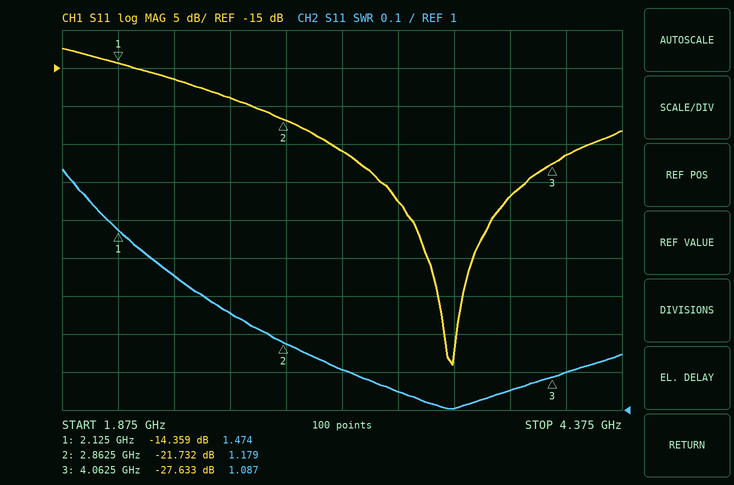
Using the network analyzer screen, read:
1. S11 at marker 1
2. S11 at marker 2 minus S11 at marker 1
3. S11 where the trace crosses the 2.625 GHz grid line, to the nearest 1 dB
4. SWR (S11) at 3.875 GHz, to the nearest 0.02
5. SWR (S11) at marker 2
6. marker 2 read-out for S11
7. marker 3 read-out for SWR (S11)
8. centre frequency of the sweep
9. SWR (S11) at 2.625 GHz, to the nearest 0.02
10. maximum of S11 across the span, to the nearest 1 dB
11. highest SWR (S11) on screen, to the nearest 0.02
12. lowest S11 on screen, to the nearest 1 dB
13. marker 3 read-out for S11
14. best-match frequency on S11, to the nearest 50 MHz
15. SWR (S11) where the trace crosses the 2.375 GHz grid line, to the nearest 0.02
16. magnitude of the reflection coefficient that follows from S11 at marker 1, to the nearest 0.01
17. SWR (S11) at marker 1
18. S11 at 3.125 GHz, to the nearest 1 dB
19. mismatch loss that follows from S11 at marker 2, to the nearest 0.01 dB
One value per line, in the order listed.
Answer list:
-14.359 dB
-7.373 dB
-19 dB
1.06
1.179
-21.732 dB
1.087
3.125 GHz
1.26
-12 dB
1.64
-54 dB
-27.633 dB
3.60 GHz
1.36
0.19
1.474
-26 dB
0.03 dB
